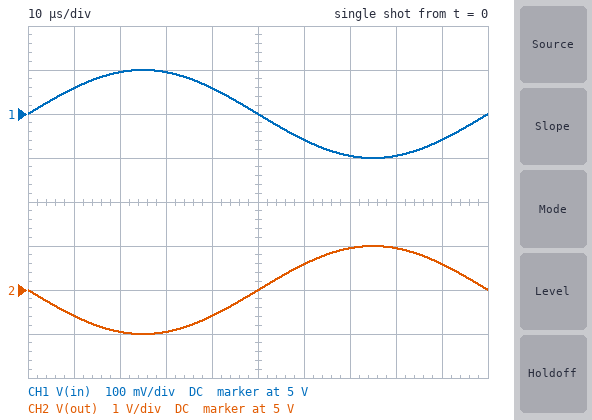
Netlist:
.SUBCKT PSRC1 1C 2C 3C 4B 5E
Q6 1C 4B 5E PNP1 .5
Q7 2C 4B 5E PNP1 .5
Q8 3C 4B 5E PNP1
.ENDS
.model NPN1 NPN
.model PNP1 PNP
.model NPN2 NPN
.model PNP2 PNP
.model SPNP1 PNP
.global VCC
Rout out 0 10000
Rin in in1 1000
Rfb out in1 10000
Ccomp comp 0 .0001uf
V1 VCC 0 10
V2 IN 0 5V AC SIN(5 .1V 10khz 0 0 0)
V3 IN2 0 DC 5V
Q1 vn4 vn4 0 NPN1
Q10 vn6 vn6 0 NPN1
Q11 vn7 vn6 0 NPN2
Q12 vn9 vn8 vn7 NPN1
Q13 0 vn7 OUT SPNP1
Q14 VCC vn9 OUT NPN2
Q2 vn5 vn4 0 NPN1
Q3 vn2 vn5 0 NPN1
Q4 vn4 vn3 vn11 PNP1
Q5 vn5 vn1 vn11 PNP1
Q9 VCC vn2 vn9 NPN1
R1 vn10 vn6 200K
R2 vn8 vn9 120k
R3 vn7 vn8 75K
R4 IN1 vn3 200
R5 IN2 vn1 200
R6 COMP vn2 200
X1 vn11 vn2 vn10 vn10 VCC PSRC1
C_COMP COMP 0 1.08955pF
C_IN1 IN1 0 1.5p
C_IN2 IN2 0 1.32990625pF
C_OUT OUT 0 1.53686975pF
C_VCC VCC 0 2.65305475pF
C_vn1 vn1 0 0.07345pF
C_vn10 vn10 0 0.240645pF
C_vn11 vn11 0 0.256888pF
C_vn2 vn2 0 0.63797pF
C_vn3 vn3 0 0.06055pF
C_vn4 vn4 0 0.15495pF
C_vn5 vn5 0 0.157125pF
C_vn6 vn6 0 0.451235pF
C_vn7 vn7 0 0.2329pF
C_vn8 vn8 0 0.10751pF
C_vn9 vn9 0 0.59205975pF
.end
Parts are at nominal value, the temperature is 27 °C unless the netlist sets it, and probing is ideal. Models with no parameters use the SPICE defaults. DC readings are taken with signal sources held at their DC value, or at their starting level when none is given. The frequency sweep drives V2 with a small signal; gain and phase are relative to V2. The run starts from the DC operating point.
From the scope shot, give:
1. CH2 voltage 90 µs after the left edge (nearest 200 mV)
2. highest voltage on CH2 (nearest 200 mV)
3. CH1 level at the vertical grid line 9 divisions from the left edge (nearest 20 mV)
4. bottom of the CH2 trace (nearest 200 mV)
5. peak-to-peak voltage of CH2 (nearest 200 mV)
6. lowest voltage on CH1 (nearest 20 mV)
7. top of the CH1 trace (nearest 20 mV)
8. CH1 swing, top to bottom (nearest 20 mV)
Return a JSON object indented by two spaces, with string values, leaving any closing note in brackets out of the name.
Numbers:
{
  "CH2 voltage 90 µs after the left edge": "5.6 V",
  "highest voltage on CH2": "6.0 V",
  "CH1 level at the vertical grid line 9 divisions from the left edge": "4.94 V",
  "bottom of the CH2 trace": "4.0 V",
  "peak-to-peak voltage of CH2": "2.0 V",
  "lowest voltage on CH1": "4.90 V",
  "top of the CH1 trace": "5.10 V",
  "CH1 swing, top to bottom": "200 mV"
}
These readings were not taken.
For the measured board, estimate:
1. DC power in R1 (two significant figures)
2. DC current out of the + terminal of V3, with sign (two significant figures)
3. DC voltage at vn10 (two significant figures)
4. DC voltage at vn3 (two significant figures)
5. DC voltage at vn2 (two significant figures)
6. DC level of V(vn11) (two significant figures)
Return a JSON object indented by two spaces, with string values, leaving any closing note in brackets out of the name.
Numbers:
{
  "DC power in R1": "370 µW",
  "DC current out of the + terminal of V3, with sign": "-100 nA",
  "DC voltage at vn10": "9.3 V",
  "DC voltage at vn3": "5.0 V",
  "DC voltage at vn2": "6.5 V",
  "DC level of V(vn11)": "5.7 V"
}
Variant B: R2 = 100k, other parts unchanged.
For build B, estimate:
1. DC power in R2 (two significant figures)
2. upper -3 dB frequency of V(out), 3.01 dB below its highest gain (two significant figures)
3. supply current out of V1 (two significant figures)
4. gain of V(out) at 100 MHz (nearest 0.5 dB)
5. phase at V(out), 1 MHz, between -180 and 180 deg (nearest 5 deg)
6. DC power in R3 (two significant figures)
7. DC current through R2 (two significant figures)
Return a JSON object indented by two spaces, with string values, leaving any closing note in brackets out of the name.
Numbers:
{
  "DC power in R2": "8.3 µW",
  "upper -3 dB frequency of V(out), 3.01 dB below its highest gain": "6.6 MHz",
  "supply current out of V1": "2.2 mA",
  "gain of V(out) at 100 MHz": "-10.5 dB",
  "phase at V(out), 1 MHz, between -180 and 180 deg": "170 deg",
  "DC power in R3": "6.0 µW",
  "DC current through R2": "9.1 µA"
}
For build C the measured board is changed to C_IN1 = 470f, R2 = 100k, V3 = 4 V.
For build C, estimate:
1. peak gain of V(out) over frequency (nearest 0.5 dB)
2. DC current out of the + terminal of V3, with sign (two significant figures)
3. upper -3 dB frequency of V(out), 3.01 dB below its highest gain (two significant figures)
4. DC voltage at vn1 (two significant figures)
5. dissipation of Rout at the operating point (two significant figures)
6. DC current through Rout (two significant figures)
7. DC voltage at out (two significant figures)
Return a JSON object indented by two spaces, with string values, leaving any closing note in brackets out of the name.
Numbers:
{
  "peak gain of V(out) over frequency": "-41.5 dB",
  "DC current out of the + terminal of V3, with sign": "-210 nA",
  "upper -3 dB frequency of V(out), 3.01 dB below its highest gain": "290 MHz",
  "DC voltage at vn1": "4.0 V",
  "dissipation of Rout at the operating point": "58 µW",
  "DC current through Rout": "76 µA",
  "DC voltage at out": "760 mV"
}
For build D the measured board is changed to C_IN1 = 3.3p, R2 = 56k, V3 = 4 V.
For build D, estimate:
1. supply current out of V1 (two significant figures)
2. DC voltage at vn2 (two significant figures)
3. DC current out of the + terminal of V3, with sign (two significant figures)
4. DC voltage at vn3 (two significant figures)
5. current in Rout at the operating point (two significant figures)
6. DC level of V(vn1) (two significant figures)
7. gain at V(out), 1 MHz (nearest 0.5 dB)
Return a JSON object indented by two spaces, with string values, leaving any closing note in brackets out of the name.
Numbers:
{
  "supply current out of V1": "85 µA",
  "DC voltage at vn2": "29 mV",
  "DC current out of the + terminal of V3, with sign": "-210 nA",
  "DC voltage at vn3": "4.6 V",
  "current in Rout at the operating point": "76 µA",
  "DC level of V(vn1)": "4.0 V",
  "gain at V(out), 1 MHz": "-41.5 dB"
}
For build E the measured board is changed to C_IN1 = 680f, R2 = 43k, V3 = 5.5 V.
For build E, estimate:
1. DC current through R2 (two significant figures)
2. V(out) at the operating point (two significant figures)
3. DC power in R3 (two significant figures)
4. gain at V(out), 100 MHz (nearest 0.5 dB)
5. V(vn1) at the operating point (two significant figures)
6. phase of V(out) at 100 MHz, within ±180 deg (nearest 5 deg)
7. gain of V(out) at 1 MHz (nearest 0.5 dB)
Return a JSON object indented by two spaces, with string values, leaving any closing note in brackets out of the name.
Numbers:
{
  "DC current through R2": "9.5 µA",
  "V(out) at the operating point": "8.5 V",
  "DC power in R3": "6.3 µW",
  "gain at V(out), 100 MHz": "-53.0 dB",
  "V(vn1) at the operating point": "5.5 V",
  "phase of V(out) at 100 MHz, within ±180 deg": "-25 deg",
  "gain of V(out) at 1 MHz": "-52.5 dB"
}
